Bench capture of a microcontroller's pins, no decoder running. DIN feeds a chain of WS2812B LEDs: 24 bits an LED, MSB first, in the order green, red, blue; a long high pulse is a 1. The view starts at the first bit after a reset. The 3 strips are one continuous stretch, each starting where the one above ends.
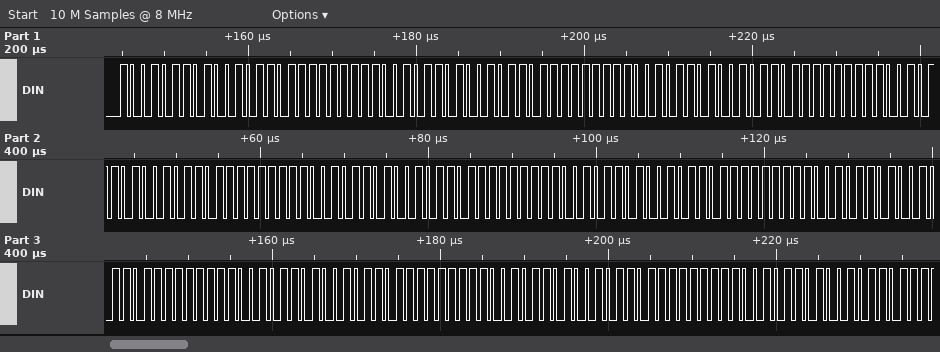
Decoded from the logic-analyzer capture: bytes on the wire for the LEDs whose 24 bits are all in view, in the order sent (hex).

96 96 FF 96 96 FF 96 96 FF 96 96 FF 96 96 FF 96 96 FF 96 96 FF 96 96 FF 96 96 FF
